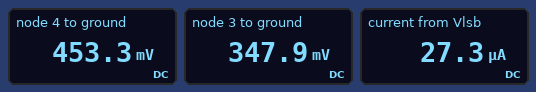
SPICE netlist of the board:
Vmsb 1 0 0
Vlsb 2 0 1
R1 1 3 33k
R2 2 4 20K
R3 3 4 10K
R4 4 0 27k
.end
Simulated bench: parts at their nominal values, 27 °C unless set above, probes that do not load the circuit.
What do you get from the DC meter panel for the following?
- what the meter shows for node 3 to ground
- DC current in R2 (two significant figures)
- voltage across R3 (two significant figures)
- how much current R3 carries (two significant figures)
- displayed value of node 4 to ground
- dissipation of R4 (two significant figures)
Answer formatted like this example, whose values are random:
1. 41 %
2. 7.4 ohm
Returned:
1. 347.9 mV
2. 27 µA
3. 110 mV
4. 11 µA
5. 453.3 mV
6. 7.6 µW
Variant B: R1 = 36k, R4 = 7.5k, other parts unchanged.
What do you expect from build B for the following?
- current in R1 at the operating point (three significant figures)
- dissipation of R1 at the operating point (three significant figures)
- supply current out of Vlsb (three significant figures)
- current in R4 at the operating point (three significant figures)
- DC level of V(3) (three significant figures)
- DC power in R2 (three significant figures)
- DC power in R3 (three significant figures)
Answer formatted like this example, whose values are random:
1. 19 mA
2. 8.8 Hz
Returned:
1. 5.30 µA
2. 1.01 µW
3. 37.8 µA
4. 32.5 µA
5. 191 mV
6. 28.6 µW
7. 281 nW
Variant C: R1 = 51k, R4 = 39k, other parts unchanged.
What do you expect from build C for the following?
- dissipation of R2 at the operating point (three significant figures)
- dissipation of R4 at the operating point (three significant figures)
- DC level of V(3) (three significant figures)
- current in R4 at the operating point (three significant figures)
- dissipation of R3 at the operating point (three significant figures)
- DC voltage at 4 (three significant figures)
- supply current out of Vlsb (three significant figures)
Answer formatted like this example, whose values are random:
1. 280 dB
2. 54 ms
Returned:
1. 10.4 µW
2. 7.57 µW
3. 454 mV
4. 13.9 µA
5. 793 nW
6. 543 mV
7. 22.8 µA
